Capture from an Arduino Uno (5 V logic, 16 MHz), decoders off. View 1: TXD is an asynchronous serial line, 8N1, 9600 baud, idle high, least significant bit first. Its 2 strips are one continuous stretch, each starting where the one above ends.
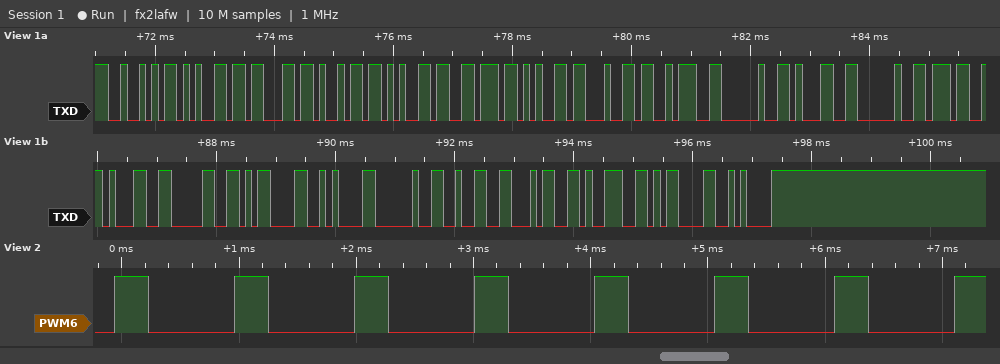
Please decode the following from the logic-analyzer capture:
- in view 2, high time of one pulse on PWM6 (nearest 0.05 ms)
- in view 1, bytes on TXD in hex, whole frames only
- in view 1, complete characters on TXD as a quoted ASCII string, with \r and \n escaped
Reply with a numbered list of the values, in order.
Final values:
1. 0.30 ms
2. 52 65 63 69 65 76 65 64 3A 20 31 20 37 31 30 0D 0A 20 32 34 39 0D 0A
3. "Recieved: 1 710\r\n 249\r\n"
